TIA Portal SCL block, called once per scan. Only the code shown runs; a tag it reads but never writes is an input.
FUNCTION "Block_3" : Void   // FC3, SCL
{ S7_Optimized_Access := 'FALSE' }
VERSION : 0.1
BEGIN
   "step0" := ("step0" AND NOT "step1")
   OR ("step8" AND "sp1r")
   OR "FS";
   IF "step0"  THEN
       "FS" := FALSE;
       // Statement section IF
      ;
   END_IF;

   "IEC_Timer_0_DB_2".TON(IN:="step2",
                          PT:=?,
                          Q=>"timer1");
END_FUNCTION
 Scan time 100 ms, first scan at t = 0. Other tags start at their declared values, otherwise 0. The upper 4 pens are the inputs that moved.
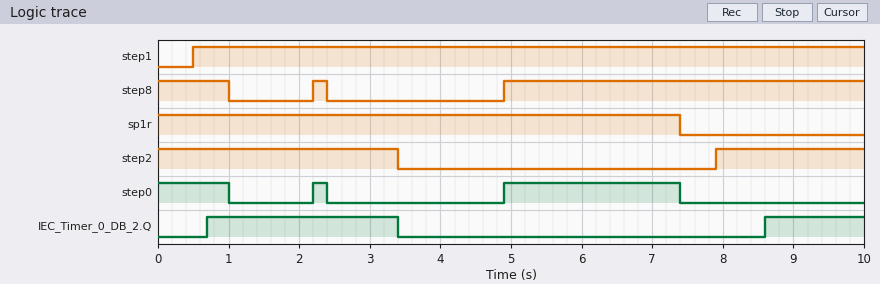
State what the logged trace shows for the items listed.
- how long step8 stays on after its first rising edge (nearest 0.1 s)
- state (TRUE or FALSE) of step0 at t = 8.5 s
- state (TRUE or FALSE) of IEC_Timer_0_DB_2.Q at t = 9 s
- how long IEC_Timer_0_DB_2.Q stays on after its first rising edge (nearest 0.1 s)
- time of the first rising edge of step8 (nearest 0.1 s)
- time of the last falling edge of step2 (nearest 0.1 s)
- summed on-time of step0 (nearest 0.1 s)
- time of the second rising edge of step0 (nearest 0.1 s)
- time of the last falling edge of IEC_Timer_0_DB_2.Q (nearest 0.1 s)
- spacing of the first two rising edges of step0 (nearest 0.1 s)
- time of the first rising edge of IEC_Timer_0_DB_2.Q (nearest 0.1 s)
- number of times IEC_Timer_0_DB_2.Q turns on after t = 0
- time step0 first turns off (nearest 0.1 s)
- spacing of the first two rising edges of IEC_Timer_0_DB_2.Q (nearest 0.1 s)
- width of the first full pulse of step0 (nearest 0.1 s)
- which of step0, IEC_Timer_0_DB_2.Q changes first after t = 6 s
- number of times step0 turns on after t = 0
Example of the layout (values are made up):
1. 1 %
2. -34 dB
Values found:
1. 0.2 s
2. FALSE
3. TRUE
4. 2.7 s
5. 2.2 s
6. 3.4 s
7. 3.7 s
8. 4.9 s
9. 3.4 s
10. 2.7 s
11. 0.7 s
12. 2
13. 1.0 s
14. 7.9 s
15. 0.2 s
16. step0
17. 2
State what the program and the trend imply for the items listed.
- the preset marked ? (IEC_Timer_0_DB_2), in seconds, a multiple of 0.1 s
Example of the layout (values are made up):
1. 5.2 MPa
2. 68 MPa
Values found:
1. 0.7 s
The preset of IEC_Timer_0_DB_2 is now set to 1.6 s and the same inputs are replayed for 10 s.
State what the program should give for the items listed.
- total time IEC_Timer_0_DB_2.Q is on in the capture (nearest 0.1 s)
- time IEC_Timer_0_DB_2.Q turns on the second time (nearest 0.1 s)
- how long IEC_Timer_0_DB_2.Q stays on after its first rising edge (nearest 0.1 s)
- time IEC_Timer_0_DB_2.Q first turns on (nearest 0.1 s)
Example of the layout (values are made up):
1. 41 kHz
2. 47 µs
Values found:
1. 2.3 s
2. 9.5 s
3. 1.8 s
4. 1.6 s
